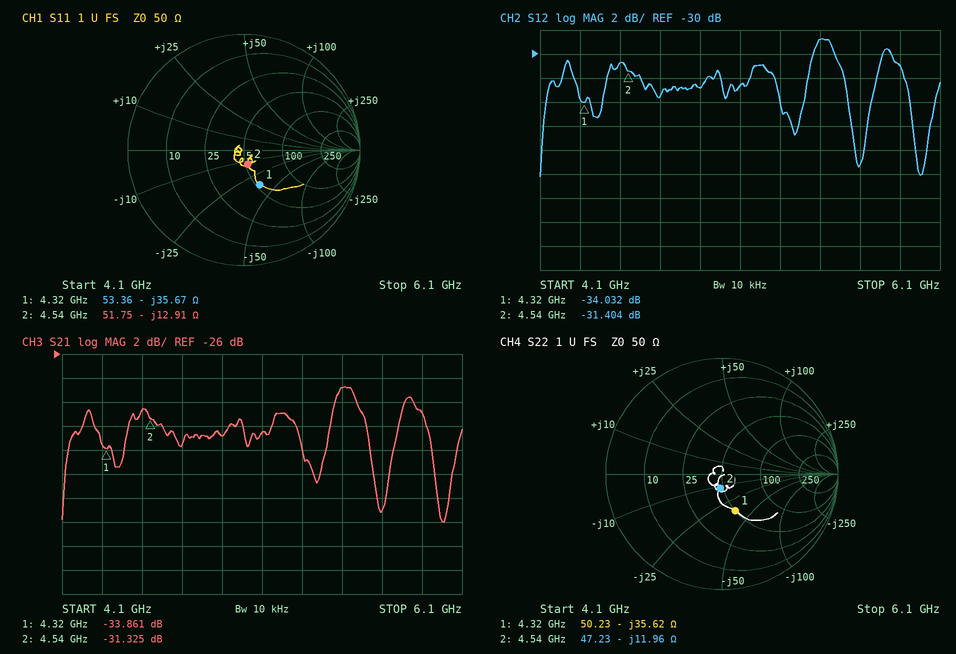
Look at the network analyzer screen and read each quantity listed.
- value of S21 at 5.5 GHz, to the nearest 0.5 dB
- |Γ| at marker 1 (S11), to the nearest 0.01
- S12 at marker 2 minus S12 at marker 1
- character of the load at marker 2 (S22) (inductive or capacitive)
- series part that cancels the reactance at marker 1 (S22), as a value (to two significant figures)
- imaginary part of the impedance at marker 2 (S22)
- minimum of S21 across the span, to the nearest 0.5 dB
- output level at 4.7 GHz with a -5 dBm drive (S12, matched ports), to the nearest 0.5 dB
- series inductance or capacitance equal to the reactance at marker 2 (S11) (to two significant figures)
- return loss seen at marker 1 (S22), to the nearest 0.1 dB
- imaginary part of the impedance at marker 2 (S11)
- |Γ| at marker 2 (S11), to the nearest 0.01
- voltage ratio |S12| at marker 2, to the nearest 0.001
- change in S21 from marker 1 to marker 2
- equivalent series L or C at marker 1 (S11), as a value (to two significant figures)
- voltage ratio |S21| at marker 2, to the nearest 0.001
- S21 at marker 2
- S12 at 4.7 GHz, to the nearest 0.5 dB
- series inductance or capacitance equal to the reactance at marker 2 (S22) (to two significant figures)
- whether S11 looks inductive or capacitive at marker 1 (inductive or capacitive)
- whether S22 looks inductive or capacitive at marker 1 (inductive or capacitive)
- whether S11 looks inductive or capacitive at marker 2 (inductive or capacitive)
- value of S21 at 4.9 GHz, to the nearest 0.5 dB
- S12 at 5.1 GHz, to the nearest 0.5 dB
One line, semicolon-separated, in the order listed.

-29.0 dB; 0.33; 2.628 dB; capacitive; 1.3 nH; -11.96 Ω; -40.0 dB; -38.5 dBm; 2.7 pF; 9.5 dB; -12.91 Ω; 0.13; 0.027; 2.536 dB; 1.0 pF; 0.027; -31.325 dB; -33.5 dB; 2.9 pF; capacitive; capacitive; capacitive; -33.0 dB; -32.5 dB
